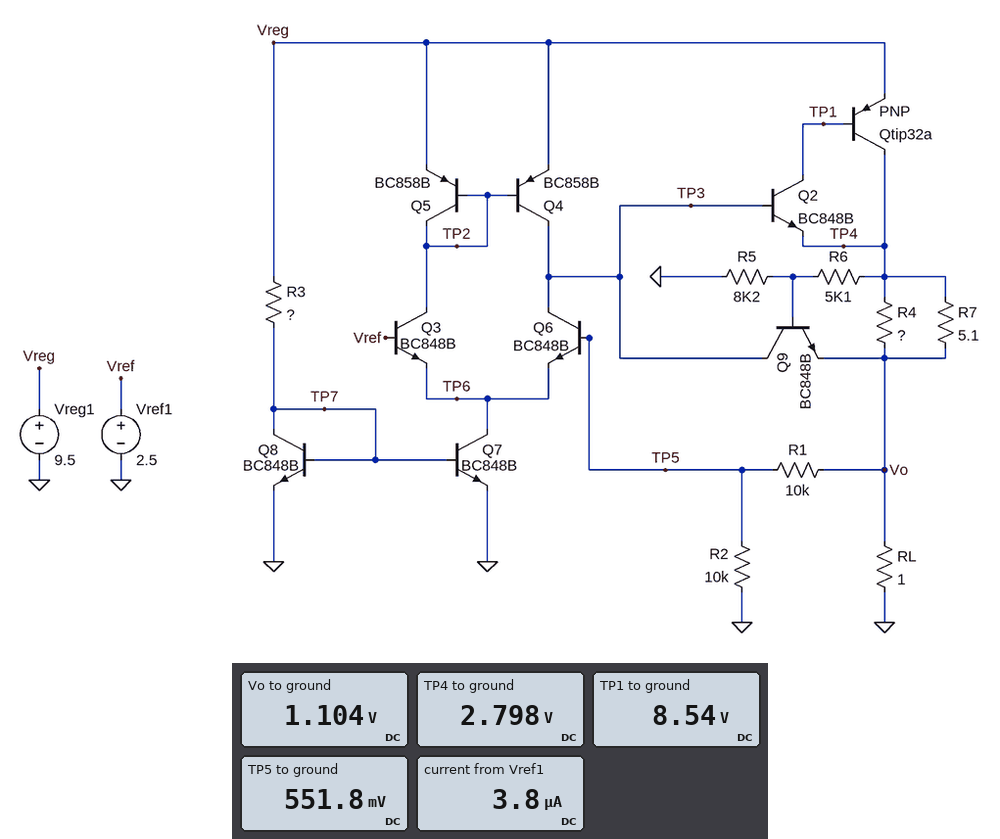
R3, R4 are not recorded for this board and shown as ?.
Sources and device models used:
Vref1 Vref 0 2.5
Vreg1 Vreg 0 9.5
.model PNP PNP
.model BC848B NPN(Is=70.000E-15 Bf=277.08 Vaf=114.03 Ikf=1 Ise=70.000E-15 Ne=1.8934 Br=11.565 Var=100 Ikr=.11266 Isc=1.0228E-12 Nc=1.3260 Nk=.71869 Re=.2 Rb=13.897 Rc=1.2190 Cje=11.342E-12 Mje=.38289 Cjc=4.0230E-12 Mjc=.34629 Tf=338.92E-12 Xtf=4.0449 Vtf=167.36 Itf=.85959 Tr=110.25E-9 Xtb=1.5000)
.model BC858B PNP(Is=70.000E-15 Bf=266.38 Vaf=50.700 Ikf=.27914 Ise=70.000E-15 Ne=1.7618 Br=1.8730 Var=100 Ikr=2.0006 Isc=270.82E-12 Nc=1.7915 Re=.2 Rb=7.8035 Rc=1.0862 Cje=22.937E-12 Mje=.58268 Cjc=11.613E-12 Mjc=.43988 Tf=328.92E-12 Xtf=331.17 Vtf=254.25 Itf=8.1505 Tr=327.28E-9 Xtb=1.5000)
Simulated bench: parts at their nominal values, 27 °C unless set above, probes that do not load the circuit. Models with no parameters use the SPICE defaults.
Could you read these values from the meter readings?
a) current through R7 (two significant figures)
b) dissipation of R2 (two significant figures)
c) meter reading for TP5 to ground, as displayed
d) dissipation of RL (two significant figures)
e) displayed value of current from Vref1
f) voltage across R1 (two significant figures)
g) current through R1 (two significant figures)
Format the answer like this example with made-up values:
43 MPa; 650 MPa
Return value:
330 mA; 30 µW; 551.8 mV; 1.2 W; 3.8 µA; 550 mV; 55 µA
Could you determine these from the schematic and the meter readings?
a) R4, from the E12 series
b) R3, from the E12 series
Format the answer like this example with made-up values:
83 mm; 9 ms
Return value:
2.2 Ω; 8.2 kΩ
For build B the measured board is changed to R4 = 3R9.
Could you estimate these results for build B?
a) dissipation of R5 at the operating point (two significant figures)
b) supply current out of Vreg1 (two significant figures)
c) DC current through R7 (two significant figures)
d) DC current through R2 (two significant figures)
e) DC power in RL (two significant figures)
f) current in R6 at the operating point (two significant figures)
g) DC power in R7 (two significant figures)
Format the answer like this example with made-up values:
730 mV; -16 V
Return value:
190 µW; 640 mA; 280 mA; 32 µA; 410 mW; 160 µA; 390 mW
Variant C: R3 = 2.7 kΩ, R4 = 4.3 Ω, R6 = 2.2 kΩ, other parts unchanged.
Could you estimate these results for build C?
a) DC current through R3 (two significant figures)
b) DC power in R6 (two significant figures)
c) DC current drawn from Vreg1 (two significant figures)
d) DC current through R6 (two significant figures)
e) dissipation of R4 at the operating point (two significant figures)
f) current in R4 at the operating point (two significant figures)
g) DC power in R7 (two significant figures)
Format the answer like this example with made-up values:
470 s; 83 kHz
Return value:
3.3 mA; 44 µW; 420 mA; 140 µA; 210 mW; 220 mA; 180 mW
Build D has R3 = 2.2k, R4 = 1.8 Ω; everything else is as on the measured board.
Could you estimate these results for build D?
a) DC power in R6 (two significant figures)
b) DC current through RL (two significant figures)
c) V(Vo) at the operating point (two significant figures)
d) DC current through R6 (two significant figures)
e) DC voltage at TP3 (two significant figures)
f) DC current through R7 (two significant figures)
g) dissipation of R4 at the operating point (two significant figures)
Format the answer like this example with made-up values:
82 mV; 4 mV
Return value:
420 µW; 1.6 A; 1.6 V; 290 µA; 4.4 V; 410 mA; 2.5 W
